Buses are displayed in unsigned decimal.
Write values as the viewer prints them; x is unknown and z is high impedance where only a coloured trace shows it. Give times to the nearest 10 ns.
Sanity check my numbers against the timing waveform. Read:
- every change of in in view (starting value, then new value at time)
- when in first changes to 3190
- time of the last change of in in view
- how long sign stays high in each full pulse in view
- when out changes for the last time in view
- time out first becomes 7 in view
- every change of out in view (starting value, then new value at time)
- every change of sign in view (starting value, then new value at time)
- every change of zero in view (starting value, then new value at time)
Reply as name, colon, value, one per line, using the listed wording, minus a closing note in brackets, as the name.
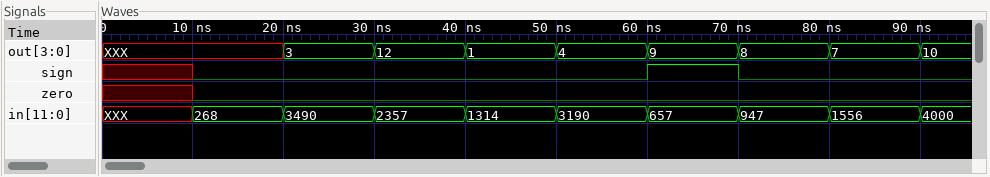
every change of in in view: XXX, 268 at 10 ns, 3490 at 20 ns, 2357 at 30 ns, 1314 at 40 ns, 3190 at 50 ns, 657 at 60 ns, 947 at 70 ns, 1556 at 80 ns, 4000 at 90 ns
when in first changes to 3190: 50 ns
time of the last change of in in view: 90 ns
how long sign stays high in each full pulse in view: 10 ns
when out changes for the last time in view: 90 ns
time out first becomes 7 in view: 80 ns
every change of out in view: XXX, 3 at 20 ns, 12 at 30 ns, 1 at 40 ns, 4 at 50 ns, 9 at 60 ns, 8 at 70 ns, 7 at 80 ns, 10 at 90 ns
every change of sign in view: x, 0 at 10 ns, 1 at 60 ns, 0 at 70 ns
every change of zero in view: x, 0 at 10 ns
